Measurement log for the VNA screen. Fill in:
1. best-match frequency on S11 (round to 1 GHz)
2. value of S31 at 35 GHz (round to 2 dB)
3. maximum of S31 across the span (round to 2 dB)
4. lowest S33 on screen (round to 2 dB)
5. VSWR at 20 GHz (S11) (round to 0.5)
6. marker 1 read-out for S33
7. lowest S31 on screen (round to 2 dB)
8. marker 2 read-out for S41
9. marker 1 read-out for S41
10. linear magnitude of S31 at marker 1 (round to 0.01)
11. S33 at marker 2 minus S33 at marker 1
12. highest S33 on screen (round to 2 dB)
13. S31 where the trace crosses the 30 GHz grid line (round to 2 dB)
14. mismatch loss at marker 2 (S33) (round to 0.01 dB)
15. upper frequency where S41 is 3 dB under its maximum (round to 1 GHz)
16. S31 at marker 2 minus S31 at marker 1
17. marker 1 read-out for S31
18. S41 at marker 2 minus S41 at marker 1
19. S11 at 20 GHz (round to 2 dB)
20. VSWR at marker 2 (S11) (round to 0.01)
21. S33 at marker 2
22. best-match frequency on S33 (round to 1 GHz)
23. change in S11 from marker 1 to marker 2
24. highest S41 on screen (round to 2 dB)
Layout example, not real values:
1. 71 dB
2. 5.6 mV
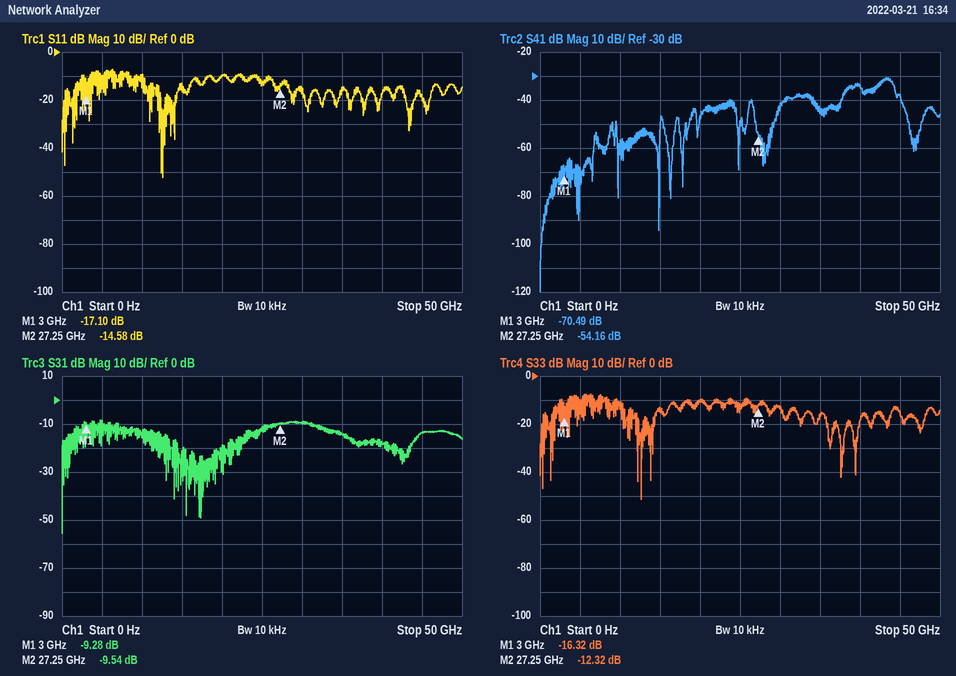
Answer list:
1. 13 GHz
2. -14 dB
3. -8 dB
4. -52 dB
5. 2.0
6. -16.32 dB
7. -56 dB
8. -54.16 dB
9. -70.49 dB
10. 0.34
11. 4.00 dB
12. -8 dB
13. -10 dB
14. 0.26 dB
15. 44 GHz
16. -0.26 dB
17. -9.28 dB
18. 16.33 dB
19. -10 dB
20. 1.46
21. -12.32 dB
22. 13 GHz
23. 2.52 dB
24. -30 dB
